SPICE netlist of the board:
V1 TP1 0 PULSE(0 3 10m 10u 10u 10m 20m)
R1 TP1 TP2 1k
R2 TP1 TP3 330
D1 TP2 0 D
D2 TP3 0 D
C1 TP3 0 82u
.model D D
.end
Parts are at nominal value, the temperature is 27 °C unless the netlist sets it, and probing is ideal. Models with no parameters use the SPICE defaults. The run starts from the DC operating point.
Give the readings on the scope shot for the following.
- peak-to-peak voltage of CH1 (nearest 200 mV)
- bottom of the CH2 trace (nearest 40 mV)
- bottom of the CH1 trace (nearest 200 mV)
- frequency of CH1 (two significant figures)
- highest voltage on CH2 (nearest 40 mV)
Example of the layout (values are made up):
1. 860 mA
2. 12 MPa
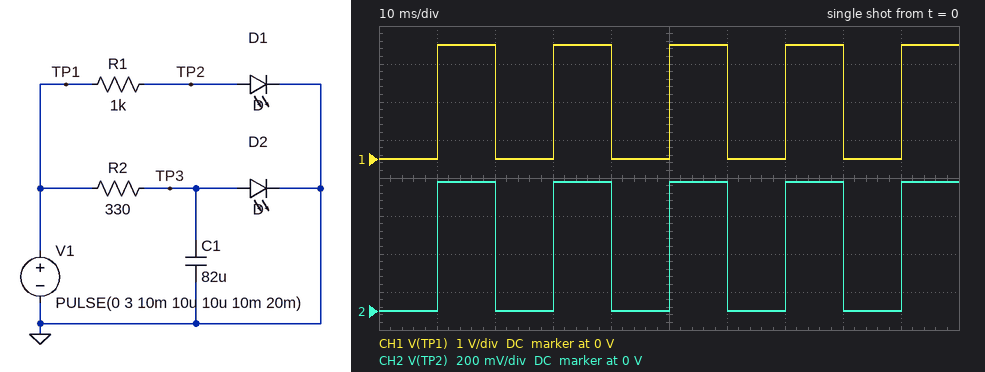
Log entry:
1. 3.0 V
2. 0 V
3. 0 V
4. 50 Hz
5. 680 mV
